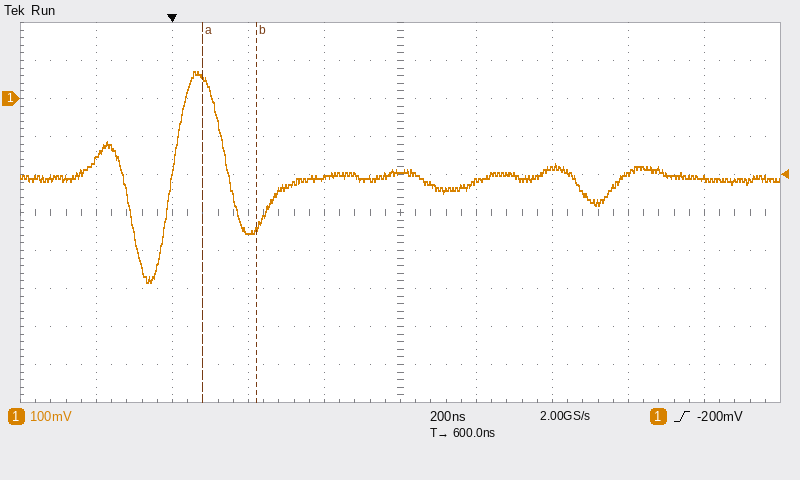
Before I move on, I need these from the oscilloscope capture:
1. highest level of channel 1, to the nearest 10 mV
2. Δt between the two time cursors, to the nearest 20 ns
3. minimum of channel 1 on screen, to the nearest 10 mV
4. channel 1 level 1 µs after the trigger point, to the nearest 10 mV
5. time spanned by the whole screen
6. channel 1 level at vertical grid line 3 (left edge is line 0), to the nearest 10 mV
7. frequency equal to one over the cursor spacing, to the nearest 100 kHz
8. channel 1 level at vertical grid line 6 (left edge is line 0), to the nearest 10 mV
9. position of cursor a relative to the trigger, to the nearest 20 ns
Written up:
70 mV
140 ns
-480 mV
-180 mV
2 µs
-350 mV
7.1 MHz
-220 mV
+80 ns
